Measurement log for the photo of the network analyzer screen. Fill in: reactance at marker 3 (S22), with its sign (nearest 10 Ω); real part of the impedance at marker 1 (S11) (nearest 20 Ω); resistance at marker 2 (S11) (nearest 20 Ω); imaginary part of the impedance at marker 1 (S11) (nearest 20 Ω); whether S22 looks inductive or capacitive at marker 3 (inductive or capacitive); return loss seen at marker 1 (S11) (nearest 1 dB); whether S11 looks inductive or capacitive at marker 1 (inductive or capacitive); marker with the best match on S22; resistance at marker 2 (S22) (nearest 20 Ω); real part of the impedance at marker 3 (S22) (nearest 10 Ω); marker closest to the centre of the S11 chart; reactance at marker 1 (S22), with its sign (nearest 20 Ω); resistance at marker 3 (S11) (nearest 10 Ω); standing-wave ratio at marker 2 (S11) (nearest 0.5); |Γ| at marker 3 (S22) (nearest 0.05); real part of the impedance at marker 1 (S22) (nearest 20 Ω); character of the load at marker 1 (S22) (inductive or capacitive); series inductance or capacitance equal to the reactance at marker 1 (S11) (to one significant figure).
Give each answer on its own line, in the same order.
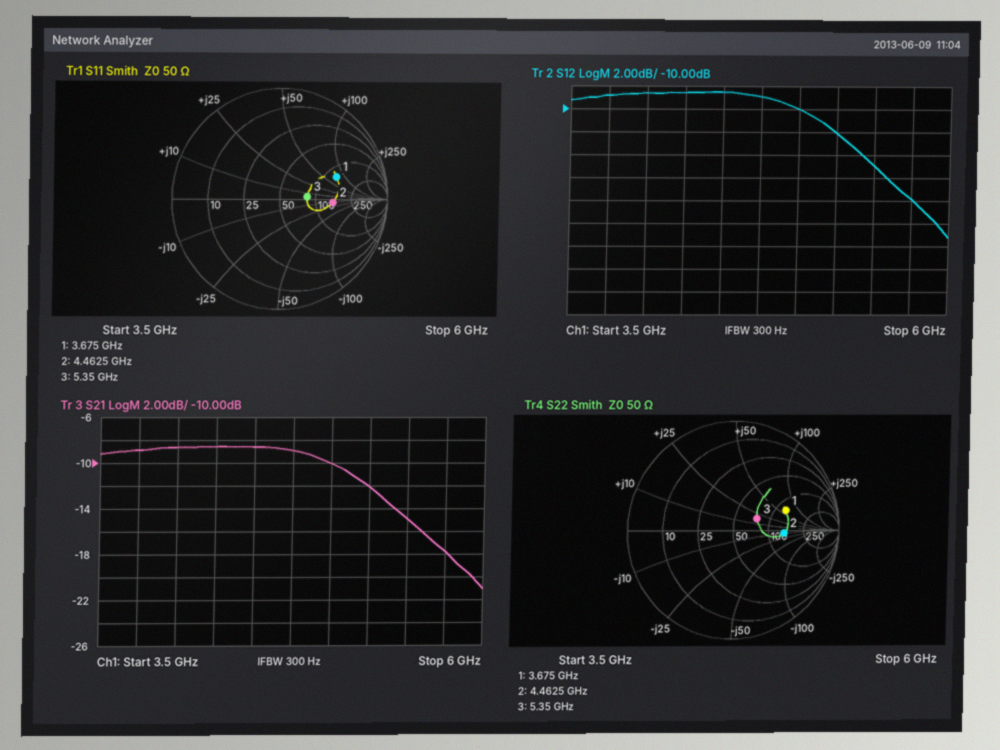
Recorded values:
+20 Ω
120 Ω
140 Ω
+80 Ω
inductive
5 dB
inductive
marker 3
140 Ω
80 Ω
marker 3
+60 Ω
80 Ω
3.0
0.25
120 Ω
inductive
3 nH
